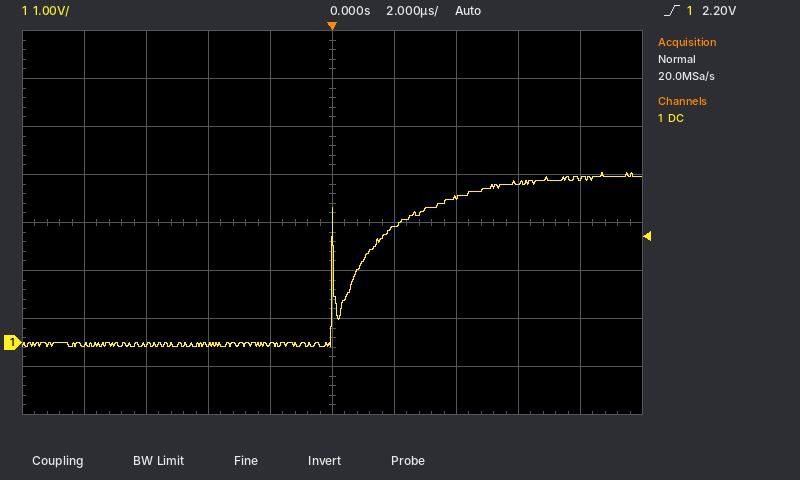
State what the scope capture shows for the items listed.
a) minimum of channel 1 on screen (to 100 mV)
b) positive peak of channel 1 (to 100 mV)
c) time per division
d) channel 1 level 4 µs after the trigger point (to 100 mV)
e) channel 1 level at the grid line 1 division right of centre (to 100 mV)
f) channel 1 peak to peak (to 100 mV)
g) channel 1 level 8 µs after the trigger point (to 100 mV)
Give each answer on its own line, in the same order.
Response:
-100 mV
3.5 V
2 µs
3.0 V
2.4 V
3.6 V
3.4 V
